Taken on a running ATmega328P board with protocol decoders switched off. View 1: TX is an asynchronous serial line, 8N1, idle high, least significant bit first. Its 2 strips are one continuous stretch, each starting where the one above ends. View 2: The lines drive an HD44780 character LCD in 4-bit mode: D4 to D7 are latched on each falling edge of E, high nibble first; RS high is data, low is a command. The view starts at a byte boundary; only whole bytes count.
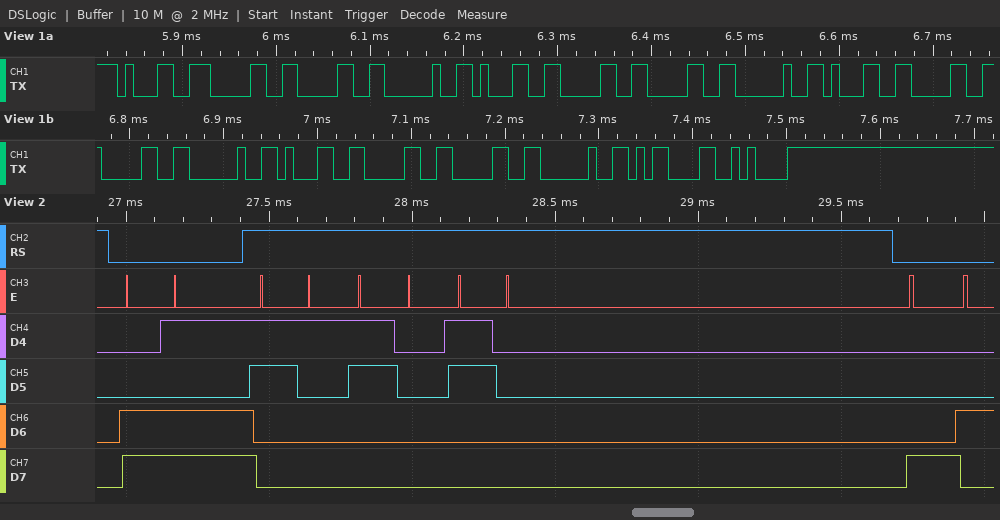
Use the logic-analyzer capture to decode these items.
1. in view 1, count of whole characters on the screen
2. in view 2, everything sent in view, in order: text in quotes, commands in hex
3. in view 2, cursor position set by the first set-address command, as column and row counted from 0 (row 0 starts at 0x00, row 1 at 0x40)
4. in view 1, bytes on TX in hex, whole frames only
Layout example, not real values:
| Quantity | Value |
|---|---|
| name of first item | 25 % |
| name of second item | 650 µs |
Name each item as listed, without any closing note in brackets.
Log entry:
| Quantity | Value |
|---|---|
| in view 1, count of whole characters on the screen | 18 |
| in view 2, everything sent in view, in order: text in quotes, commands in hex | 0xCD "100" 0x84 |
| in view 2, cursor position set by the first set-address command, as column and row counted from 0 | column 13, row 1 |
| in view 1, bytes on TX in hex, whole frames only | 31 30 30 20 31 30 30 20 31 30 30 20 31 30 30 20 0D 0A |
